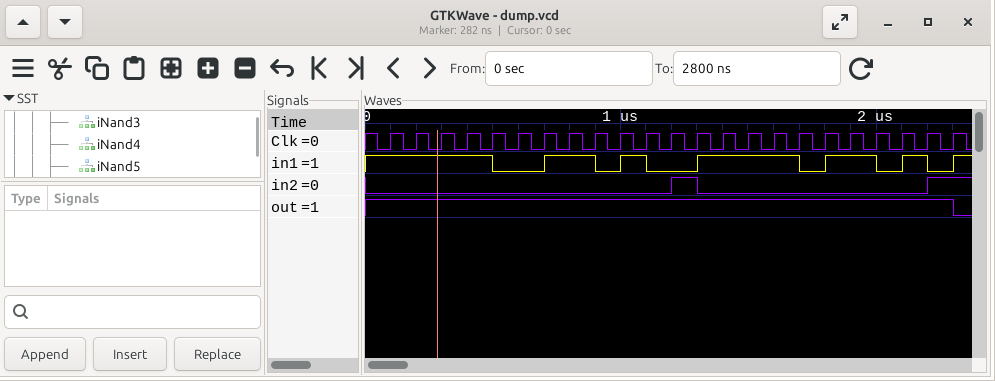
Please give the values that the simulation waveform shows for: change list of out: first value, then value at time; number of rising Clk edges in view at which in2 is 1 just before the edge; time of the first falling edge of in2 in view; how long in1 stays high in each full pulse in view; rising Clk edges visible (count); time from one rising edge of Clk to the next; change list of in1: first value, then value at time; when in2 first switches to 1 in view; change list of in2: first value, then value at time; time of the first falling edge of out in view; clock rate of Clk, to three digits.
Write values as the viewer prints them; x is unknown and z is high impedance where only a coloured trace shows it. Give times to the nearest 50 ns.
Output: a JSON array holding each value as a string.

["1, 0 at 2300 ns", "2", "1300 ns", "200 ns, 100 ns, 400 ns, 200 ns, 100 ns", "23", "100 ns", "1, 0 at 500 ns, 1 at 700 ns, 0 at 900 ns, 1 at 1000 ns, 0 at 1100 ns, 1 at 1300 ns, 0 at 1700 ns, 1 at 1800 ns, 0 at 2000 ns, 1 at 2100 ns, 0 at 2200 ns, 1 at 2300 ns", "1200 ns", "0, 1 at 1200 ns, 0 at 1300 ns, 1 at 2200 ns", "2300 ns", "10.0 MHz"]
